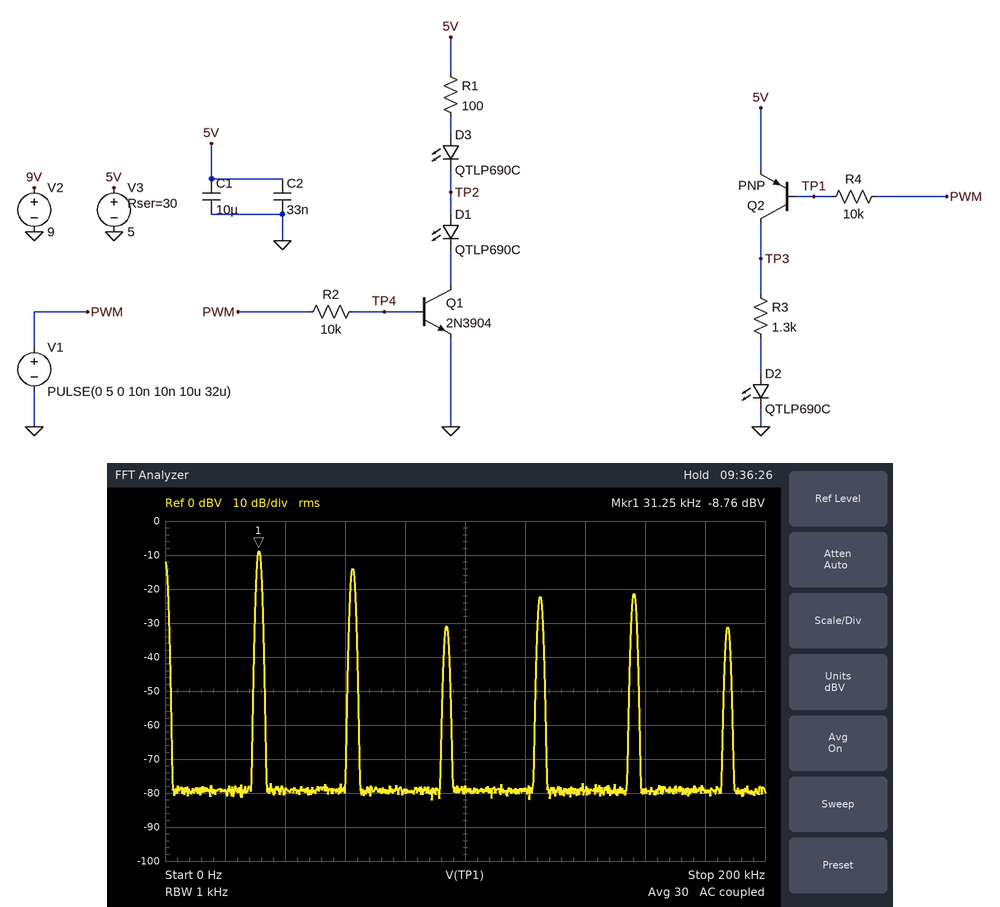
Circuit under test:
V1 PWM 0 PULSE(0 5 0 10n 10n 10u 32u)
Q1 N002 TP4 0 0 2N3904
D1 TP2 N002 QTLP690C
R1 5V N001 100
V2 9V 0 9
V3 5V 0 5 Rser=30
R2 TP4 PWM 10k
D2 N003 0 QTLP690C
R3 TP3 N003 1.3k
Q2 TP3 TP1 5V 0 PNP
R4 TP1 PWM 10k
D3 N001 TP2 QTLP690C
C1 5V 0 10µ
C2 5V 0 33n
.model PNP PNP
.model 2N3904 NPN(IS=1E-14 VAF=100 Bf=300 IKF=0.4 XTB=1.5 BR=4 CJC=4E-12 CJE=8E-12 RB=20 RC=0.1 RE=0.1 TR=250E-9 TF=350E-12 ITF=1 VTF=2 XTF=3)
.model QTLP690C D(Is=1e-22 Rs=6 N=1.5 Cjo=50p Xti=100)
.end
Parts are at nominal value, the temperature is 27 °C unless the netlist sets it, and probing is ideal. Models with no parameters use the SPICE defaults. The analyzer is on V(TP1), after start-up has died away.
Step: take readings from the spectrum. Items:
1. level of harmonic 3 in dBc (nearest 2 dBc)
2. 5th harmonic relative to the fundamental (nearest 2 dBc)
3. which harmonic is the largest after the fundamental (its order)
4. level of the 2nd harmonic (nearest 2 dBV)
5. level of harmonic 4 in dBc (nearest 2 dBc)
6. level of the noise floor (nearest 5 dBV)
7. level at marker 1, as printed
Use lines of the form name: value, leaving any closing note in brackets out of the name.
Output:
level of harmonic 3 in dBc: -22 dBc
5th harmonic relative to the fundamental: -12 dBc
which harmonic is the largest after the fundamental: 2
level of the 2nd harmonic: -14 dBV
level of harmonic 4 in dBc: -14 dBc
level of the noise floor: -80 dBV
level at marker 1, as printed: -8.76 dBV
